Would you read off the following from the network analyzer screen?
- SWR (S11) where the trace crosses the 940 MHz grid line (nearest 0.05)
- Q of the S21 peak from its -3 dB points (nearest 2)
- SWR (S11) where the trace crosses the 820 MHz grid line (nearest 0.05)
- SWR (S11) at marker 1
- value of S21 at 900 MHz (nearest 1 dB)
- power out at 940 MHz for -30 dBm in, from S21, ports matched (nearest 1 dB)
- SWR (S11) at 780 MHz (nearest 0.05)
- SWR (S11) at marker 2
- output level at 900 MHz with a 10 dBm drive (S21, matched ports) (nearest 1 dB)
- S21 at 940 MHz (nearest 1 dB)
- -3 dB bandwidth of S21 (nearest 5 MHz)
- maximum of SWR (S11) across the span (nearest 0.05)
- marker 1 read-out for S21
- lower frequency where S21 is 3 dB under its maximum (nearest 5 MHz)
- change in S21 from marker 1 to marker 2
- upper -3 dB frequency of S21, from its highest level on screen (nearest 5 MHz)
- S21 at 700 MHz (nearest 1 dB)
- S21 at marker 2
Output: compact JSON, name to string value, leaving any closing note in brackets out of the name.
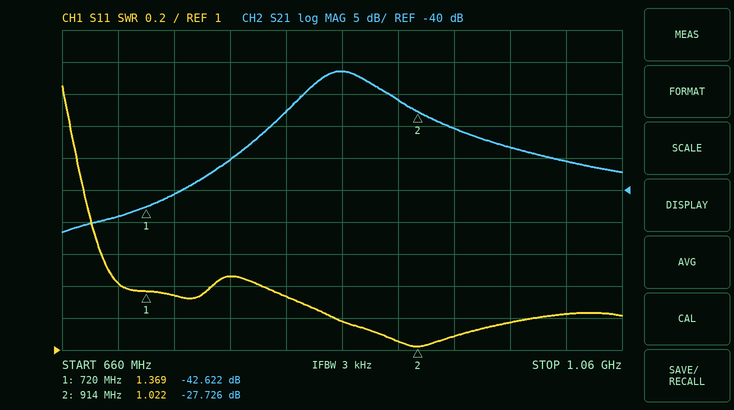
{"SWR (S11) where the trace crosses the 940 MHz grid line": "1.10", "Q of the S21 peak from its -3 dB points": "16", "SWR (S11) where the trace crosses the 820 MHz grid line": "1.35", "SWR (S11) at marker 1": "1.369", "value of S21 at 900 MHz": "-26 dB", "power out at 940 MHz for -30 dBm in, from S21, ports matched": "-60 dBm", "SWR (S11) at 780 MHz": "1.45", "SWR (S11) at marker 2": "1.022", "output level at 900 MHz with a 10 dBm drive (S21, matched ports)": "-16 dBm", "S21 at 940 MHz": "-30 dB", "-3 dB bandwidth of S21": "55 MHz", "maximum of SWR (S11) across the span": "2.65", "marker 1 read-out for S21": "-42.622 dB", "lower frequency where S21 is 3 dB under its maximum": "835 MHz", "change in S21 from marker 1 to marker 2": "14.896 dB", "upper -3 dB frequency of S21, from its highest level on screen": "890 MHz", "S21 at 700 MHz": "-44 dB", "S21 at marker 2": "-27.726 dB"}
